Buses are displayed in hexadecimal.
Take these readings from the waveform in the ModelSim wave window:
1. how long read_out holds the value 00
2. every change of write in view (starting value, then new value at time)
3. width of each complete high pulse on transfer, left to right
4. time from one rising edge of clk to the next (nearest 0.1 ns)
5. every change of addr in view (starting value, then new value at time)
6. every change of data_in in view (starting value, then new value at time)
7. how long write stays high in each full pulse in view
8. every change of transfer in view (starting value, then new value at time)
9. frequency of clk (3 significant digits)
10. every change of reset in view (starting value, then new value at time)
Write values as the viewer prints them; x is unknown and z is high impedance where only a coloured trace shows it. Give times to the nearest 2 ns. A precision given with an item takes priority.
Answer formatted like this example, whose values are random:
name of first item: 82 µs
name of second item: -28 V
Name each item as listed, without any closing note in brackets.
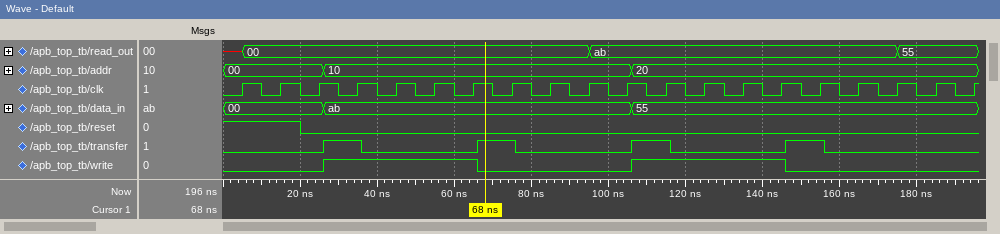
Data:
how long read_out holds the value 00: 90 ns
every change of write in view: 0, 1 at 26 ns, 0 at 66 ns, 1 at 106 ns, 0 at 146 ns
width of each complete high pulse on transfer, left to right: 10 ns, 10 ns, 10 ns, 10 ns
time from one rising edge of clk to the next: 10 ns
every change of addr in view: 00, 10 at 26 ns, 20 at 106 ns
every change of data_in in view: 00, ab at 26 ns, 55 at 106 ns
how long write stays high in each full pulse in view: 40 ns, 40 ns
every change of transfer in view: 0, 1 at 26 ns, 0 at 36 ns, 1 at 66 ns, 0 at 76 ns, 1 at 106 ns, 0 at 116 ns, 1 at 146 ns, 0 at 156 ns
frequency of clk: 100 MHz
every change of reset in view: 1, 0 at 20 ns
